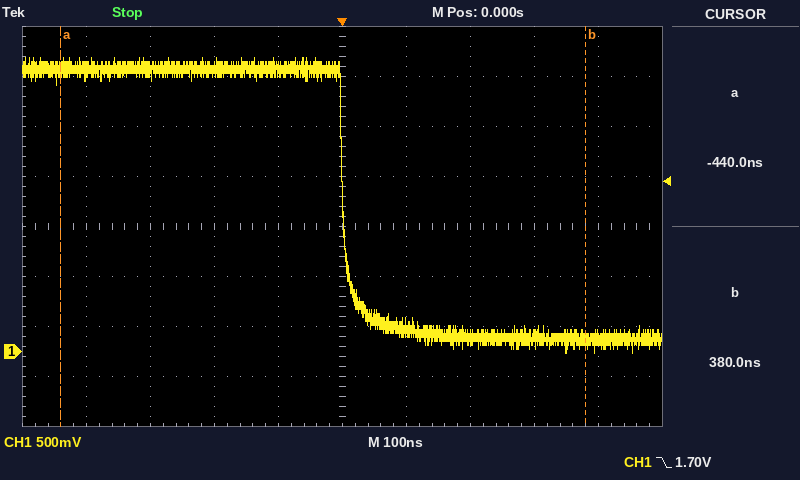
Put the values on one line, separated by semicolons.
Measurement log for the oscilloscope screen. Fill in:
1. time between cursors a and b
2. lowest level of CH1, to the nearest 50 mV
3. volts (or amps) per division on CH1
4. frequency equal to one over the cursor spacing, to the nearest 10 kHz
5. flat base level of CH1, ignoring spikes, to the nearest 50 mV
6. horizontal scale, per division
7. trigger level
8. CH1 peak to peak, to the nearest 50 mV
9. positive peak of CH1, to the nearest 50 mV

820 ns; 0 mV; 500 mV; 1.22 MHz; 150 mV; 100 ns; 1.70 V; 2.95 V; 2.95 V
